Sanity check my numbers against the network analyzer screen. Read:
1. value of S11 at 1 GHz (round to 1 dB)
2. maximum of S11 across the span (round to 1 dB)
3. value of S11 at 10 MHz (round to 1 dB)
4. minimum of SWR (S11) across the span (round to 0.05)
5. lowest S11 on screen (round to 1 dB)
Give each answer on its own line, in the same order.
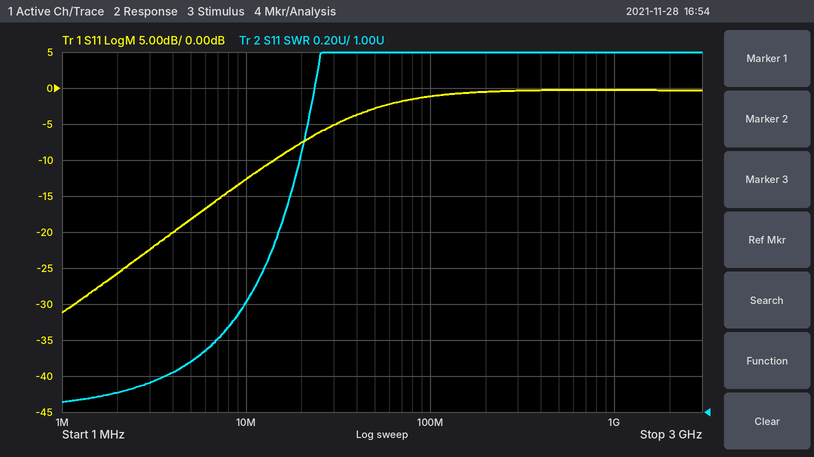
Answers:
0 dB
0 dB
-13 dB
1.05
-31 dB
